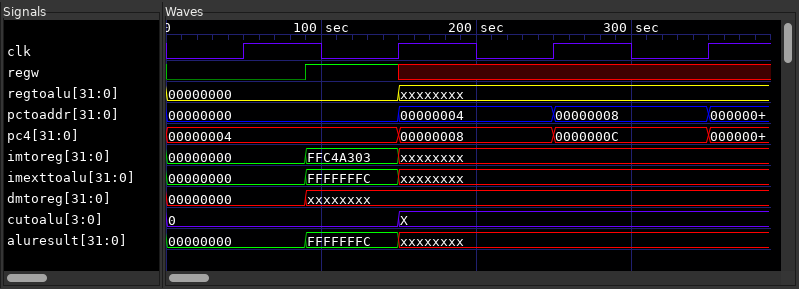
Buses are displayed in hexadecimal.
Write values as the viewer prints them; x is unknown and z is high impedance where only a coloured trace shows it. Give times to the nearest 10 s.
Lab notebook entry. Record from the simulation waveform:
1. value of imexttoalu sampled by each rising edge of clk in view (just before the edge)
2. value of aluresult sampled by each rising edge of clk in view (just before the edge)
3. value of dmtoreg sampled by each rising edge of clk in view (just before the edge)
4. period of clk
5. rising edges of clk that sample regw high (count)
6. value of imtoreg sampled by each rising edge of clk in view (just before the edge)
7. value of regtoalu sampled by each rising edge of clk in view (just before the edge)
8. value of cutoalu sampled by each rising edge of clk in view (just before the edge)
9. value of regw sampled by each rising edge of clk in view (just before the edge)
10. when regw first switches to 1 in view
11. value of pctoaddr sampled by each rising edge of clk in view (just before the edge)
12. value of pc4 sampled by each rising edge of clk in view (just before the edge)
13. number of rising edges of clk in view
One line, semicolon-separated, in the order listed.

00000000, FFFFFFFC, xxxxxxxx, xxxxxxxx; 00000000, FFFFFFFC, xxxxxxxx, xxxxxxxx; 00000000, xxxxxxxx, xxxxxxxx, xxxxxxxx; 100 s; 1; 00000000, FFC4A303, xxxxxxxx, xxxxxxxx; 00000000, 00000000, xxxxxxxx, xxxxxxxx; 0, 0, X, X; 0 1 x x; 90 s; 00000000, 00000000, 00000004, 00000008; 00000004, 00000004, 00000008, 0000000C; 4
